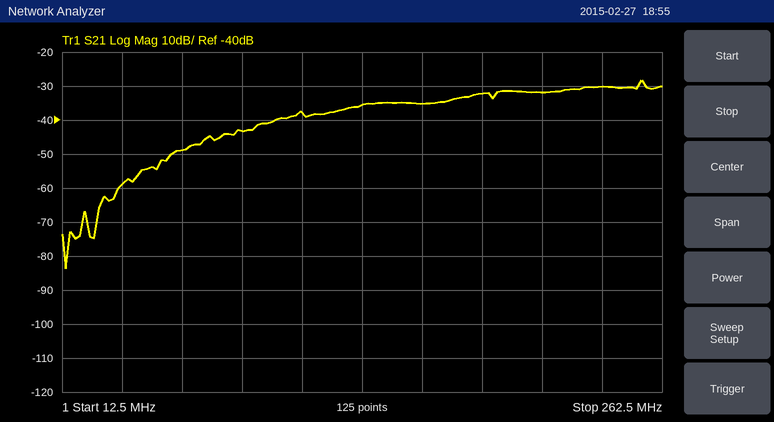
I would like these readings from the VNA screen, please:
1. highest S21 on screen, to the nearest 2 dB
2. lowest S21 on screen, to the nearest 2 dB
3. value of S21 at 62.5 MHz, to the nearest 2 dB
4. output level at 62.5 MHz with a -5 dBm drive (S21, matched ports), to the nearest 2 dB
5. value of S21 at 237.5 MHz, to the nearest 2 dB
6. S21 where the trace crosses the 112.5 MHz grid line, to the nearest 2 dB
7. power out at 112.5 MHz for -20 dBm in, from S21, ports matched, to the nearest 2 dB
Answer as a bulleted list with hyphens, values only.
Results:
- -28 dB
- -84 dB
- -48 dB
- -54 dBm
- -30 dB
- -38 dB
- -58 dBm
